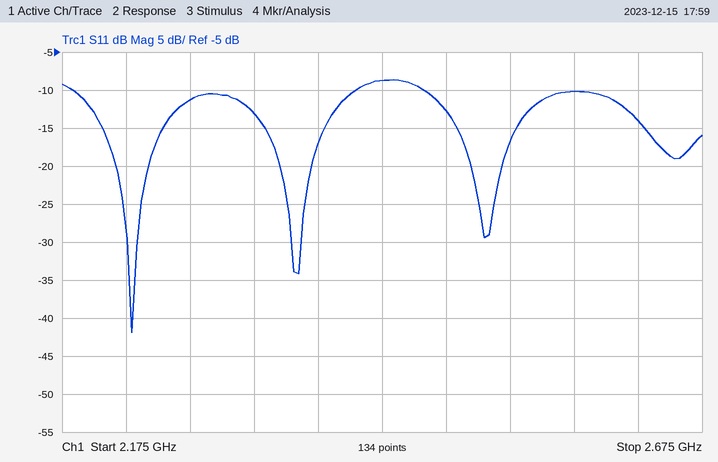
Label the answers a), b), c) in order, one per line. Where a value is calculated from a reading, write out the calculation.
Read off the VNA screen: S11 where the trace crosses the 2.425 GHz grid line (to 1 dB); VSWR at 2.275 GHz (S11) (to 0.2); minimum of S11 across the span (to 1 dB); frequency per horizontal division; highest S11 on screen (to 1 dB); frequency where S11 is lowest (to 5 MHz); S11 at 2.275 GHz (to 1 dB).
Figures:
a) -9 dB
b) |Γ| = 10^(-11/20) = 0.2818; VSWR = (1 + 0.2818)/(1 − 0.2818) ≈ 1.8
c) -42 dB
d) 50 MHz
e) -9 dB
f) 2.230 GHz
g) -11 dB
